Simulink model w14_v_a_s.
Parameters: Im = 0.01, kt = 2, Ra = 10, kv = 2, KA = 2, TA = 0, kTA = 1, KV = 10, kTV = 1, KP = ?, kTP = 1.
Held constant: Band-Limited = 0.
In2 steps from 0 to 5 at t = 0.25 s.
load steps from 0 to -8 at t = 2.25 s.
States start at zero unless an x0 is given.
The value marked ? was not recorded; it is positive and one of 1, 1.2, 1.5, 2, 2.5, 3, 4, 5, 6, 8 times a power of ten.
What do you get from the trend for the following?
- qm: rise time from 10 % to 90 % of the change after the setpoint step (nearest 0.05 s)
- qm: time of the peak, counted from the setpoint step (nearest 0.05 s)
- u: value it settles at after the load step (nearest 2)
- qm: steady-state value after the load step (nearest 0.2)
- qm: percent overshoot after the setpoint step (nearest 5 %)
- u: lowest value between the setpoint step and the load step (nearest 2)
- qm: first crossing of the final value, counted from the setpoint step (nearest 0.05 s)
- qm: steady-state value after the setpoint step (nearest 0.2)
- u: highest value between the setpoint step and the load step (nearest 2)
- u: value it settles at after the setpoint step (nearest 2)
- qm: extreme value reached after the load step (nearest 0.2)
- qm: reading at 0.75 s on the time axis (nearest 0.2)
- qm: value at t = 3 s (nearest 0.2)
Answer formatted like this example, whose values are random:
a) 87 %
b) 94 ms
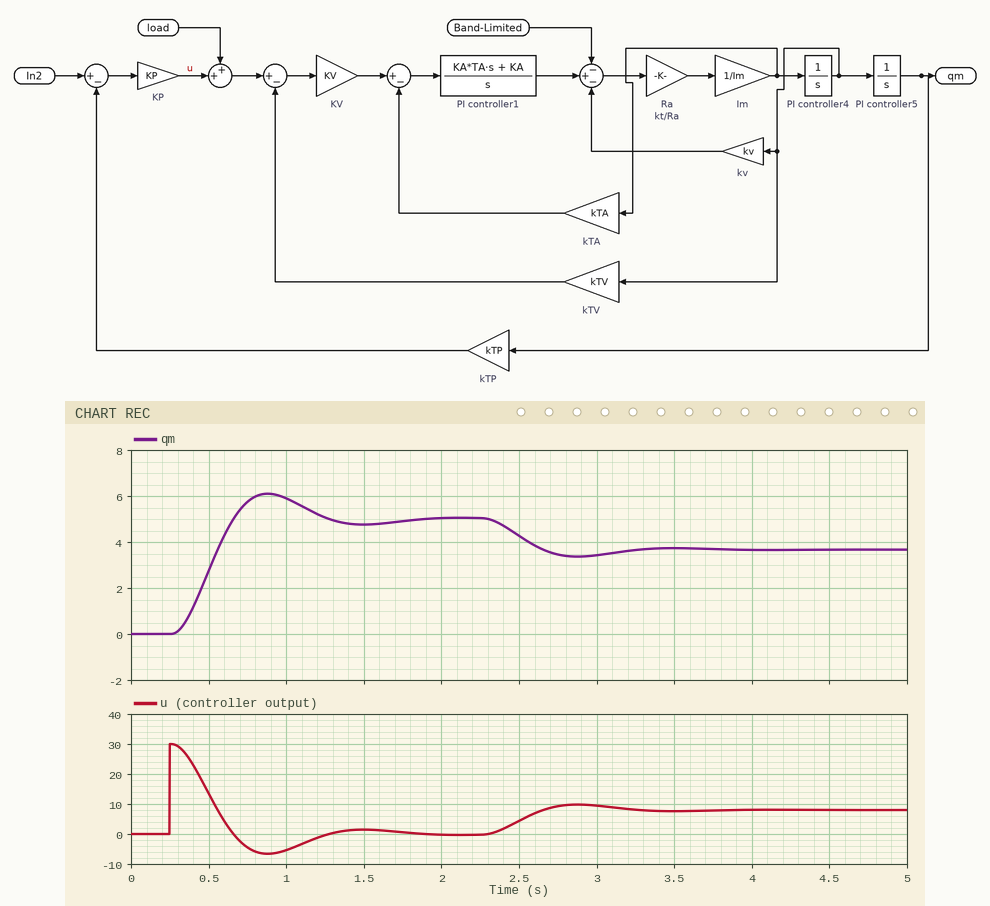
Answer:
a) 0.25 s
b) 0.65 s
c) 8
d) 3.6
e) 20 %
f) -6
g) 0.40 s
h) 5.0
i) 30
j) 0
k) 3.4
l) 5.8
m) 3.4
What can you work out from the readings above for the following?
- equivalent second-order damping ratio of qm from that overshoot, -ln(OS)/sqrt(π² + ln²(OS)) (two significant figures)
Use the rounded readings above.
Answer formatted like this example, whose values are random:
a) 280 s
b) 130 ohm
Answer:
a) 0.46
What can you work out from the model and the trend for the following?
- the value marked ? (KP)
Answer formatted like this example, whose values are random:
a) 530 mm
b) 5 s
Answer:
a) 6
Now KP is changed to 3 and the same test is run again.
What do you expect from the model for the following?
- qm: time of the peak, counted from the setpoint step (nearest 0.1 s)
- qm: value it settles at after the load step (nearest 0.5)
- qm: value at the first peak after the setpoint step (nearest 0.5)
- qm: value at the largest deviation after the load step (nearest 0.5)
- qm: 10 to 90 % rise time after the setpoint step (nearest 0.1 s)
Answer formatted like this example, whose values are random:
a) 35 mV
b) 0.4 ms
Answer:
a) 1.0 s
b) 2.5
c) 5.5
d) 2.0
e) 0.5 s
